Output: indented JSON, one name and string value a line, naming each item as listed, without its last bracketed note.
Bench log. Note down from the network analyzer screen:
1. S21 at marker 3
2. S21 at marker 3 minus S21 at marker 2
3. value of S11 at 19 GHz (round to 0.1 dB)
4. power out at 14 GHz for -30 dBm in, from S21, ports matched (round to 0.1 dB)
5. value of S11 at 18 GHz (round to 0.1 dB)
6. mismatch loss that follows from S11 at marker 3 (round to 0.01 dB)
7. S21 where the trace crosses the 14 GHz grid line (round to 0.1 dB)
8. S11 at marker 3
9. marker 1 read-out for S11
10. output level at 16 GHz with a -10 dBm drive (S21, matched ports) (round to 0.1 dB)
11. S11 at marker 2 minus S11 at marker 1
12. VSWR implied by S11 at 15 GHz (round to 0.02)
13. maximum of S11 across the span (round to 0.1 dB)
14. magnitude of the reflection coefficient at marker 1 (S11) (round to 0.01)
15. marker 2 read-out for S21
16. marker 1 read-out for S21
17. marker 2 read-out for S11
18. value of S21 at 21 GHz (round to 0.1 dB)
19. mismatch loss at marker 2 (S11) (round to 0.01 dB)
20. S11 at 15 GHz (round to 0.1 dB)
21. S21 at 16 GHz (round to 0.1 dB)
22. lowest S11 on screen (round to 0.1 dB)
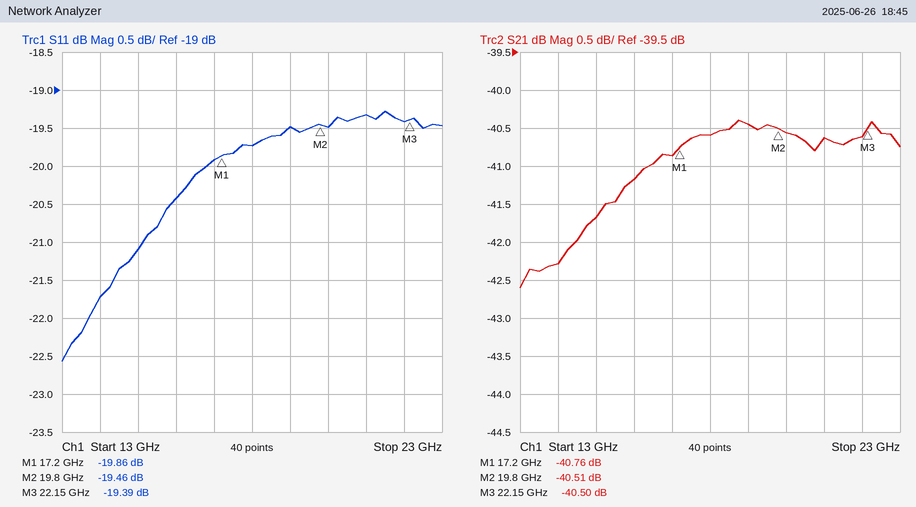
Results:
{
  "S21 at marker 3": "-40.50 dB",
  "S21 at marker 3 minus S21 at marker 2": "0.01 dB",
  "value of S11 at 19 GHz": "-19.5 dB",
  "power out at 14 GHz for -30 dBm in, from S21, ports matched": "-72.3 dBm",
  "value of S11 at 18 GHz": "-19.7 dB",
  "mismatch loss that follows from S11 at marker 3": "0.05 dB",
  "S21 where the trace crosses the 14 GHz grid line": "-42.3 dB",
  "S11 at marker 3": "-19.39 dB",
  "marker 1 read-out for S11": "-19.86 dB",
  "output level at 16 GHz with a -10 dBm drive (S21, matched ports)": "-51.2 dBm",
  "S11 at marker 2 minus S11 at marker 1": "0.40 dB",
  "VSWR implied by S11 at 15 GHz": "1.20",
  "maximum of S11 across the span": "-19.3 dB",
  "magnitude of the reflection coefficient at marker 1 (S11)": "0.10",
  "marker 2 read-out for S21": "-40.51 dB",
  "marker 1 read-out for S21": "-40.76 dB",
  "marker 2 read-out for S11": "-19.46 dB",
  "value of S21 at 21 GHz": "-40.6 dB",
  "mismatch loss at marker 2 (S11)": "0.05 dB",
  "S11 at 15 GHz": "-21.1 dB",
  "S21 at 16 GHz": "-41.2 dB",
  "lowest S11 on screen": "-22.6 dB"
}
